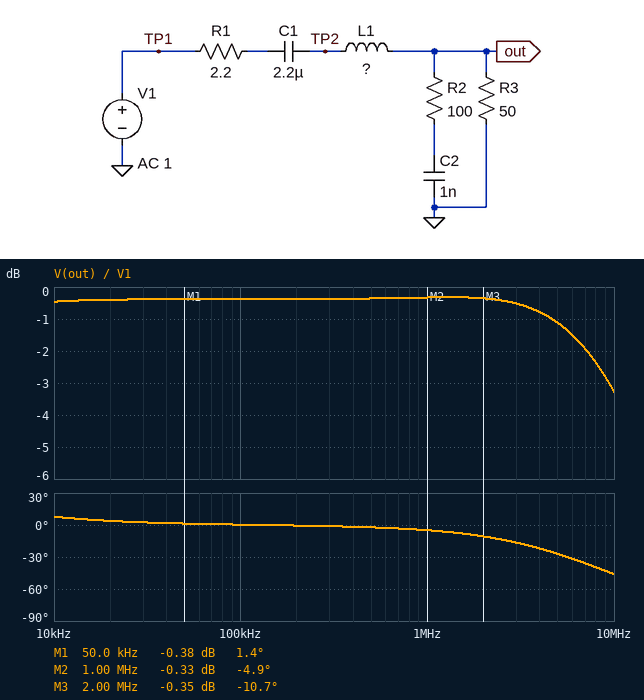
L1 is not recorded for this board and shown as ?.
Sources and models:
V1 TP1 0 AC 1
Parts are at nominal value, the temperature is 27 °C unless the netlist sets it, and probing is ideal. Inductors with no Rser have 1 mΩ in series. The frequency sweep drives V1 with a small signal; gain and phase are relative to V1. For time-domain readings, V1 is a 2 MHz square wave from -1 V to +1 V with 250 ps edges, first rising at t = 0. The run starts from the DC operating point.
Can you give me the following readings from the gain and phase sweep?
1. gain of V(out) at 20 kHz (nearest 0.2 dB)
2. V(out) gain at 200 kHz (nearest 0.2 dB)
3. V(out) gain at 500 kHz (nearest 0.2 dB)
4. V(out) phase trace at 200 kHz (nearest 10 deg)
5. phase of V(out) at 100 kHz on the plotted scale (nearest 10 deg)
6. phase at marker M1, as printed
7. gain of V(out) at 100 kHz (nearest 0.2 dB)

-0.4 dB
-0.4 dB
-0.4 dB
0 deg
0 deg
1.4 deg
-0.4 dB
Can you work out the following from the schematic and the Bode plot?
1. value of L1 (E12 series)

560 nH
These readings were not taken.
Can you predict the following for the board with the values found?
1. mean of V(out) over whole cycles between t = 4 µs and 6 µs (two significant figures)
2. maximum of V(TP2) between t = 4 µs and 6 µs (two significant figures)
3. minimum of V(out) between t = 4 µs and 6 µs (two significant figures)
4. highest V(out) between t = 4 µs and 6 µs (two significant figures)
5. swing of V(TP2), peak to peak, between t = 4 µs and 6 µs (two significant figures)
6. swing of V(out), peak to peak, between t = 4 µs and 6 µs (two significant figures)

920 mV
2.0 V
-75 mV
1.9 V
2.1 V
2.0 V
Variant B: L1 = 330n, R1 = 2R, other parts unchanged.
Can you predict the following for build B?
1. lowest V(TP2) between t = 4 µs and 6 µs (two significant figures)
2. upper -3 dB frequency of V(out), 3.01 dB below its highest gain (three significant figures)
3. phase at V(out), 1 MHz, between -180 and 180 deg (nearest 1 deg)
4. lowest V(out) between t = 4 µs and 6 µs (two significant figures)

-130 mV
16.9 MHz
-3 deg
-62 mV
